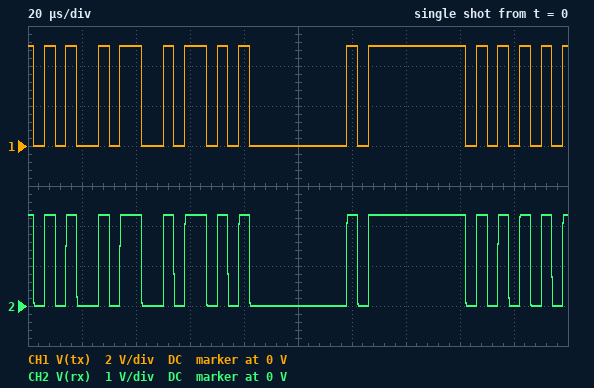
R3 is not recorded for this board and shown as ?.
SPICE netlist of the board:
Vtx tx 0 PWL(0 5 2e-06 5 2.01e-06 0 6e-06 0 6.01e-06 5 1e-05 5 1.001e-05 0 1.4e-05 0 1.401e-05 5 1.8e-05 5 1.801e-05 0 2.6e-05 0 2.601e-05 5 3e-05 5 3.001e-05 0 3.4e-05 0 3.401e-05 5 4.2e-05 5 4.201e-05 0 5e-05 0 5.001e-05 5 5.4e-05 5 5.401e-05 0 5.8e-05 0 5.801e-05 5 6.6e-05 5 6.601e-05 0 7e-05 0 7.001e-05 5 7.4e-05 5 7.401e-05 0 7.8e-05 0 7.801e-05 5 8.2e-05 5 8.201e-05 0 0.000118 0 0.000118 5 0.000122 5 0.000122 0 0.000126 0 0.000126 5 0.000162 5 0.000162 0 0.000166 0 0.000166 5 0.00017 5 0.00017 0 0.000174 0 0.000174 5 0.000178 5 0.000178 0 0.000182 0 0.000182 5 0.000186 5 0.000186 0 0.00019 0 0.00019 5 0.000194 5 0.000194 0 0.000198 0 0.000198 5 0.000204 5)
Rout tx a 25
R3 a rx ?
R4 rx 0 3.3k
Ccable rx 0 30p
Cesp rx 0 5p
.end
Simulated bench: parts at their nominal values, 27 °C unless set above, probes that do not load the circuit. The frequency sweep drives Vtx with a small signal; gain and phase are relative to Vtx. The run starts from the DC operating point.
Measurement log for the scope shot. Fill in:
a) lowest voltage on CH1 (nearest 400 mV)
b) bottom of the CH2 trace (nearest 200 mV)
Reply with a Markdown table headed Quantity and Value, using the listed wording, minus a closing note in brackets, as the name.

| Quantity | Value |
|---|---|
| lowest voltage on CH1 | 0 V |
| bottom of the CH2 trace | 0 V |
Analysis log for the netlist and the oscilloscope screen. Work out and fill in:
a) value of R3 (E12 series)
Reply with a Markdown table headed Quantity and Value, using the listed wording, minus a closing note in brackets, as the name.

| Quantity | Value |
|---|---|
| value of R3 | 3.9 kΩ |
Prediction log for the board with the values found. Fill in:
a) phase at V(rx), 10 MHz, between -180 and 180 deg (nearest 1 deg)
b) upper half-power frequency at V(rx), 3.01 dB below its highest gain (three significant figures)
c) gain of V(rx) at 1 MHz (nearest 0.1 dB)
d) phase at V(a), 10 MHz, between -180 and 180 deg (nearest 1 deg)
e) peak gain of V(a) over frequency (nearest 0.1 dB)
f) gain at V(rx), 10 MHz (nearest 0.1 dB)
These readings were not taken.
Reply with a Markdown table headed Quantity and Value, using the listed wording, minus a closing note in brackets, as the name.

| Quantity | Value |
|---|---|
| phase at V(rx), 10 MHz, between -180 and 180 deg | -76 deg |
| upper half-power frequency at V(rx), 3.01 dB below its highest gain | 2.54 MHz |
| gain of V(rx) at 1 MHz | -7.4 dB |
| phase at V(a), 10 MHz, between -180 and 180 deg | 0 deg |
| peak gain of V(a) over frequency | 0 dB |
| gain at V(rx), 10 MHz | -19.0 dB |
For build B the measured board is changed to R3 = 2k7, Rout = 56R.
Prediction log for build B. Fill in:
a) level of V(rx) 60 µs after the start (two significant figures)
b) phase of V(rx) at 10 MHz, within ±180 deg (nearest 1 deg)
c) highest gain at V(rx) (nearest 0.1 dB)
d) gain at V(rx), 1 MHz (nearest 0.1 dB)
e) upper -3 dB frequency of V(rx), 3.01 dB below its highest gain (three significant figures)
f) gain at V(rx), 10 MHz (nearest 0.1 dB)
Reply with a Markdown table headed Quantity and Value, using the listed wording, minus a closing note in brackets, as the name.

| Quantity | Value |
|---|---|
| level of V(rx) 60 µs after the start | 2.7 V |
| phase of V(rx) at 10 MHz, within ±180 deg | -73 deg |
| highest gain at V(rx) | -5.3 dB |
| gain at V(rx), 1 MHz | -5.7 dB |
| upper -3 dB frequency of V(rx), 3.01 dB below its highest gain | 3.03 MHz |
| gain at V(rx), 10 MHz | -16.0 dB |
